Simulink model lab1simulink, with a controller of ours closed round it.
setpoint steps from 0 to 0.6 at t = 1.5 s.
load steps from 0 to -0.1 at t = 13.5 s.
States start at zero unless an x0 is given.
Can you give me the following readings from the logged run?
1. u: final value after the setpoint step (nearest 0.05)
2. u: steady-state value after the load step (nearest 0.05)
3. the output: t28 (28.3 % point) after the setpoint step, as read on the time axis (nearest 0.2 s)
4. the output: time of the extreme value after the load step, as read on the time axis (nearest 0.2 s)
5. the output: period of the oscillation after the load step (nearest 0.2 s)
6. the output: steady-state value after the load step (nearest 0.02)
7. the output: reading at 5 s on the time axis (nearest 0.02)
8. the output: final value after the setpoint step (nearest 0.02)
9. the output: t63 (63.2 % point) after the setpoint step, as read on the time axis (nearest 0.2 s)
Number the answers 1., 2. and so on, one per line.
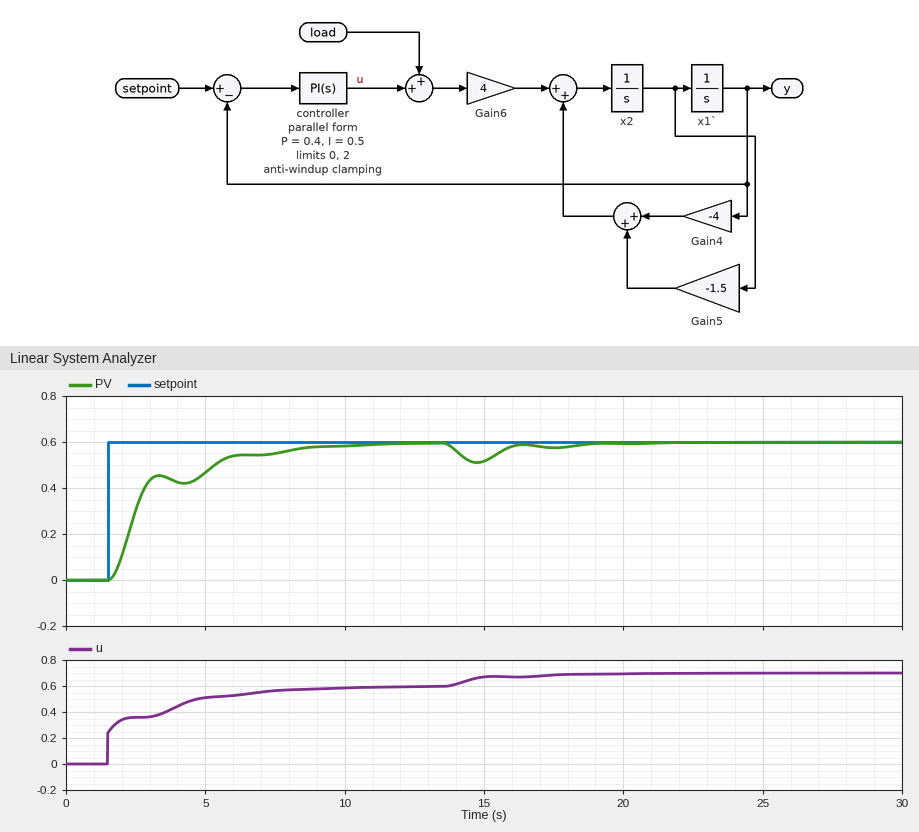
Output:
1. 0.60
2. 0.70
3. 2.2 s
4. 14.8 s
5. 2.8 s
6. 0.60
7. 0.46
8. 0.60
9. 2.8 s
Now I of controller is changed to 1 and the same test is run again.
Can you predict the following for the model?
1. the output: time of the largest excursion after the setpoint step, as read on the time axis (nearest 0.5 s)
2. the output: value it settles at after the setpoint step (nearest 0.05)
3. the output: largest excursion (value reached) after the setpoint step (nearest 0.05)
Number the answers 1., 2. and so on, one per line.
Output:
1. 6.0 s
2. 0.60
3. 0.65
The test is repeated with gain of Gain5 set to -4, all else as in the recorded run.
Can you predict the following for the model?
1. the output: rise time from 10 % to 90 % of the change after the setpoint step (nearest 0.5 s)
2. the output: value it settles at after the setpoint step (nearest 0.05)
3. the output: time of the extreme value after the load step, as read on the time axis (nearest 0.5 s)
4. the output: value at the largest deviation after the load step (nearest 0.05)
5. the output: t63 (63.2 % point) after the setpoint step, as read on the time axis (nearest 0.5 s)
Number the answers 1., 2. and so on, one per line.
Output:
1. 4.0 s
2. 0.60
3. 15.0 s
4. 0.55
5. 3.5 s
